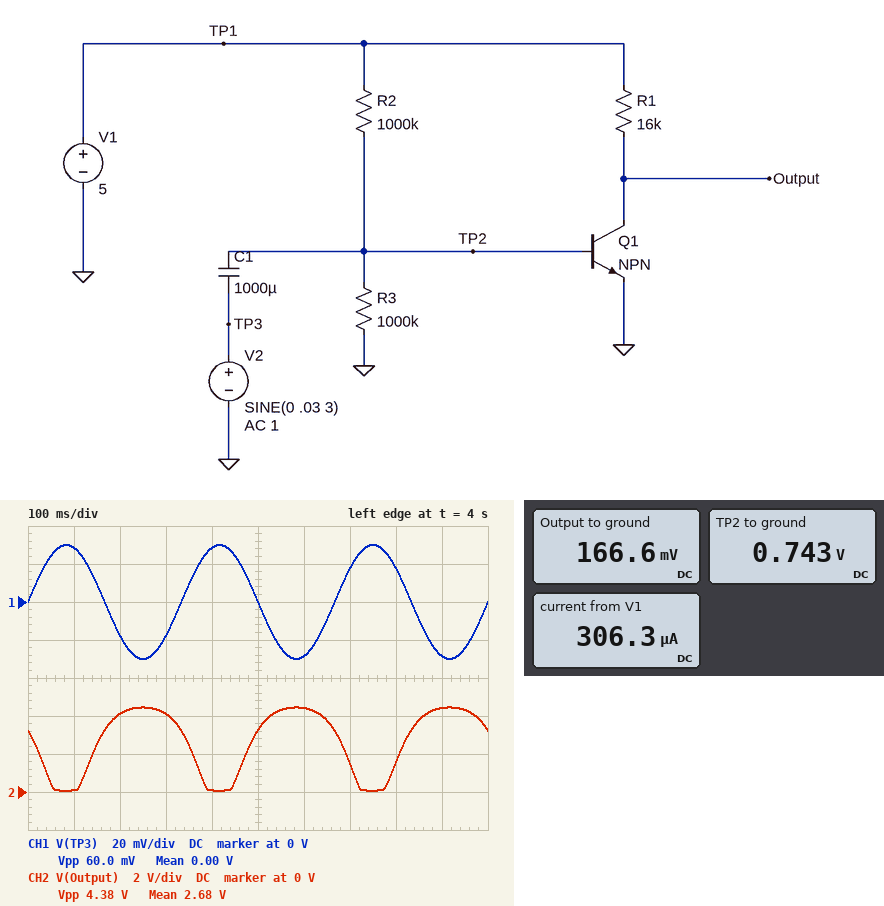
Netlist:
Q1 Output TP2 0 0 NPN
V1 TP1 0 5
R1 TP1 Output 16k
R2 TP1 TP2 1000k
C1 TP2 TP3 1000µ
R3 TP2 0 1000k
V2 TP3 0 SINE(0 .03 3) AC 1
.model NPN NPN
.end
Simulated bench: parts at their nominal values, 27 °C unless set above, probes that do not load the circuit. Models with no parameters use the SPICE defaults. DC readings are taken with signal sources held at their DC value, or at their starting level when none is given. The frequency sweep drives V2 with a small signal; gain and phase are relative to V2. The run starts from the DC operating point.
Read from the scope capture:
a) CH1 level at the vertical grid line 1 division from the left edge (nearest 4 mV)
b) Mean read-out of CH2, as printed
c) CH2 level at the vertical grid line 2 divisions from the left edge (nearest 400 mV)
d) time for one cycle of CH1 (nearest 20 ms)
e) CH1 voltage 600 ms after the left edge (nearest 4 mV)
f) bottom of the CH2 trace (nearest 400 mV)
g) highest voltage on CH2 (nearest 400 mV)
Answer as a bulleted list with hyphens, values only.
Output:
- 28 mV
- 2.68 V
- 4.0 V
- 340 ms
- -28 mV
- 0 V
- 4.4 V
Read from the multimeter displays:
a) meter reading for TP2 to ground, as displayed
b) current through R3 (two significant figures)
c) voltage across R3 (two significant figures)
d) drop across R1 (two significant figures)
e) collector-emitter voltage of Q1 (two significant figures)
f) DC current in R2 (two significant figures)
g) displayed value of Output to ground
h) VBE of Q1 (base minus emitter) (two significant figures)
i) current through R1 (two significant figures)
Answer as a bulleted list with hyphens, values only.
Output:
- 0.743 V
- 740 nA
- 740 mV
- 4.8 V
- 170 mV
- 4.3 µA
- 166.6 mV
- 740 mV
- 300 µA
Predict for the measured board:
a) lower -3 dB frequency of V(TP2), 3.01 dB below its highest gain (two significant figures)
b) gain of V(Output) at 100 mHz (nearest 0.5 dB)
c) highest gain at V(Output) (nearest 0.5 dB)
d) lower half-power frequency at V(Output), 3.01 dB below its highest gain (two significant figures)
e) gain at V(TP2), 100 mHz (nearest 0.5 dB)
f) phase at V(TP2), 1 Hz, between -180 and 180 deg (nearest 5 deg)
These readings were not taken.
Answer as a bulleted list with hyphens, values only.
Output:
- 370 mHz
- 29.5 dB
- 41.5 dB
- 370 mHz
- -11.5 dB
- 20 deg
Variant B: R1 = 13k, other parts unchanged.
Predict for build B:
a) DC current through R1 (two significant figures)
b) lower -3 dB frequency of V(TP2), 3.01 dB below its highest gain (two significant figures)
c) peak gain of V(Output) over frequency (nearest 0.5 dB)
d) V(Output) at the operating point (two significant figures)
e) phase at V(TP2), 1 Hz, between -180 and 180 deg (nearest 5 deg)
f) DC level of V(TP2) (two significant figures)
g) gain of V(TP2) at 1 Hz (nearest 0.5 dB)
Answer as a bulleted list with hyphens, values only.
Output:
- 350 µA
- 22 mHz
- 45.0 dB
- 440 mV
- 0 deg
- 750 mV
- 0 dB
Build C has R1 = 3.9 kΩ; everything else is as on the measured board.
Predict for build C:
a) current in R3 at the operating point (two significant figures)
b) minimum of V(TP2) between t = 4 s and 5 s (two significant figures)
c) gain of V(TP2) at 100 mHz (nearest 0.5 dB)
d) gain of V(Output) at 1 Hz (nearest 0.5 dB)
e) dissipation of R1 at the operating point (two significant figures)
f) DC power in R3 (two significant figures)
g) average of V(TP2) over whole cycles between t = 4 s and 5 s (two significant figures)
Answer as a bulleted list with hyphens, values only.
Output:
- 750 nA
- 710 mV
- 0 dB
- 34.5 dB
- 480 µW
- 560 nW
- 740 mV
